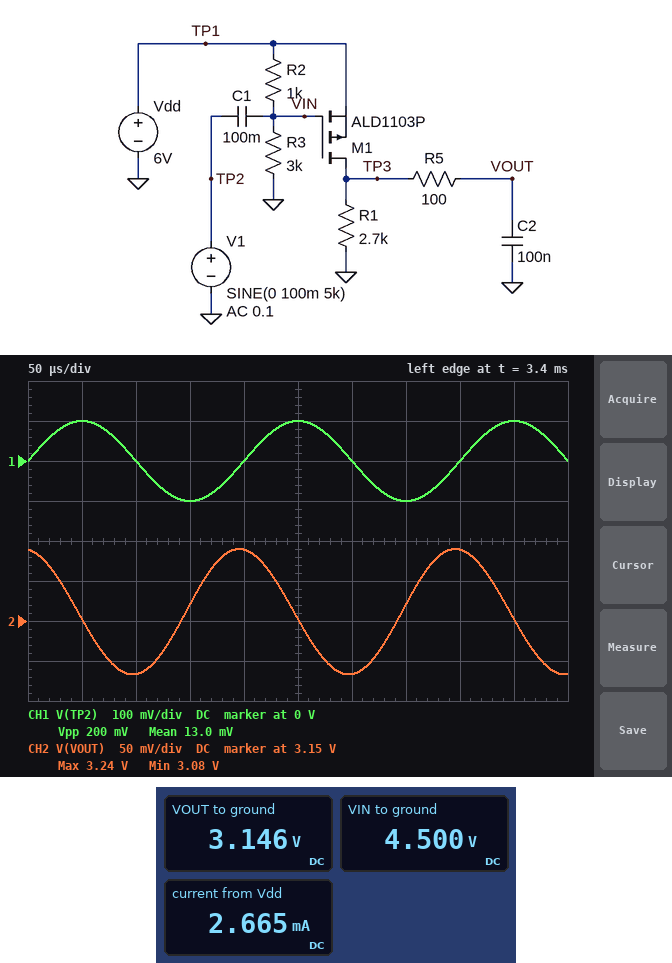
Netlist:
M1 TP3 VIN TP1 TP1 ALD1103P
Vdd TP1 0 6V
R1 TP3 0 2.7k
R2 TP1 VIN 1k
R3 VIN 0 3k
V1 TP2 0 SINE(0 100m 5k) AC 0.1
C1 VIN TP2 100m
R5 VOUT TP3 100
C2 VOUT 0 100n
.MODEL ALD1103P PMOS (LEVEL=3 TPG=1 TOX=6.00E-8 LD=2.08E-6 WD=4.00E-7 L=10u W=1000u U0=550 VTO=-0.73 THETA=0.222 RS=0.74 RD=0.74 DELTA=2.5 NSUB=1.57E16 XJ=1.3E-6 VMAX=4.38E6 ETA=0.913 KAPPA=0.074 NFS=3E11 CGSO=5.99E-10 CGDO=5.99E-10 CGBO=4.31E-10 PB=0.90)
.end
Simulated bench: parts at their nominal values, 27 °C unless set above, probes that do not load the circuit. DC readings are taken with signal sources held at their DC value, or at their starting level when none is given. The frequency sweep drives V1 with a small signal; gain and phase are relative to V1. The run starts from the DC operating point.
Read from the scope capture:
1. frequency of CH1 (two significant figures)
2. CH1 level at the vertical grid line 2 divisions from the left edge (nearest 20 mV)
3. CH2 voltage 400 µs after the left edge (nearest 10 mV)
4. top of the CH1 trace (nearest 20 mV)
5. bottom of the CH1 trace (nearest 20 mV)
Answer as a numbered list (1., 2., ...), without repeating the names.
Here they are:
1. 5.0 kHz
2. 0 V
3. 3.24 V
4. 100 mV
5. -100 mV
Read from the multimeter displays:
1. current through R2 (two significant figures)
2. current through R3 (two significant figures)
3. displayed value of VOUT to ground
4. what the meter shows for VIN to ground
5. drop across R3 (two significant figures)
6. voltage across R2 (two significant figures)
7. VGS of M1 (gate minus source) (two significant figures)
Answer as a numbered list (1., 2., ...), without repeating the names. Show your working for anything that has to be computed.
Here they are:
1. (6 V - 4.5 V) / 1 kΩ = 1.5 mA
2. (4.5 V) / 3 kΩ = 1.5 mA
3. 3.146 V
4. 4.500 V
5. 4.5 V = 4.5 V
6. 6 V - 4.5 V = 1.5 V
7. 4.5 V - 6 V = -1.5 V
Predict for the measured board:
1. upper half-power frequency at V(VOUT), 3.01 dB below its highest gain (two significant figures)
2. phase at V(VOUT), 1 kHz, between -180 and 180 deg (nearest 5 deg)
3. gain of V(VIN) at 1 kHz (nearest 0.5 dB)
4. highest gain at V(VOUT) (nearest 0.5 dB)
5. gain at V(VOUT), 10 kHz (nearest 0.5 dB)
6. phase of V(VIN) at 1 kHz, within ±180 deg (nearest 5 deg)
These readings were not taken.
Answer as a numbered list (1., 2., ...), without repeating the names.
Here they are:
1. 590 Hz
2. 120 deg
3. 0 dB
4. 16.5 dB
5. -8.0 dB
6. 0 deg
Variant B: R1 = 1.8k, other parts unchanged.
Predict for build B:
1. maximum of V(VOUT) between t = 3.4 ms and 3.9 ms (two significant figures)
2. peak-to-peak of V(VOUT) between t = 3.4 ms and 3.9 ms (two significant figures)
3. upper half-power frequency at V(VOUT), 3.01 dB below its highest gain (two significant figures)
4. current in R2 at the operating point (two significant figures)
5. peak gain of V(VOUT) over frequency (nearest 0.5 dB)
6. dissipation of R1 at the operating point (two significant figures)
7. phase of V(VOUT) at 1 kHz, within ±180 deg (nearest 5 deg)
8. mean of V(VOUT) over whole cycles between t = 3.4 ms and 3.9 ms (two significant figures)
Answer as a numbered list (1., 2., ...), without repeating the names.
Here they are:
1. 2.2 V
2. 150 mV
3. 860 Hz
4. 1.5 mA
5. 13.0 dB
6. 2.5 mW
7. 130 deg
8. 2.1 V
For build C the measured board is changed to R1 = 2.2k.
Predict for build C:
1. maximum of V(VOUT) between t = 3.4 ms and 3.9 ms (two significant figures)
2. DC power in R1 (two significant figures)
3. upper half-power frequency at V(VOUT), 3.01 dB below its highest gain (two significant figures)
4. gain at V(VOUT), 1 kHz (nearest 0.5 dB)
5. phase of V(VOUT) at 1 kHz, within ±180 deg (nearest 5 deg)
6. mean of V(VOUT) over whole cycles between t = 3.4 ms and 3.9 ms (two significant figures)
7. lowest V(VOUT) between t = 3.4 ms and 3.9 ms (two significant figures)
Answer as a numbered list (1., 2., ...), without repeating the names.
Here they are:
1. 2.7 V
2. 3.0 mW
3. 720 Hz
4. 10.0 dB
5. 125 deg
6. 2.6 V
7. 2.5 V
